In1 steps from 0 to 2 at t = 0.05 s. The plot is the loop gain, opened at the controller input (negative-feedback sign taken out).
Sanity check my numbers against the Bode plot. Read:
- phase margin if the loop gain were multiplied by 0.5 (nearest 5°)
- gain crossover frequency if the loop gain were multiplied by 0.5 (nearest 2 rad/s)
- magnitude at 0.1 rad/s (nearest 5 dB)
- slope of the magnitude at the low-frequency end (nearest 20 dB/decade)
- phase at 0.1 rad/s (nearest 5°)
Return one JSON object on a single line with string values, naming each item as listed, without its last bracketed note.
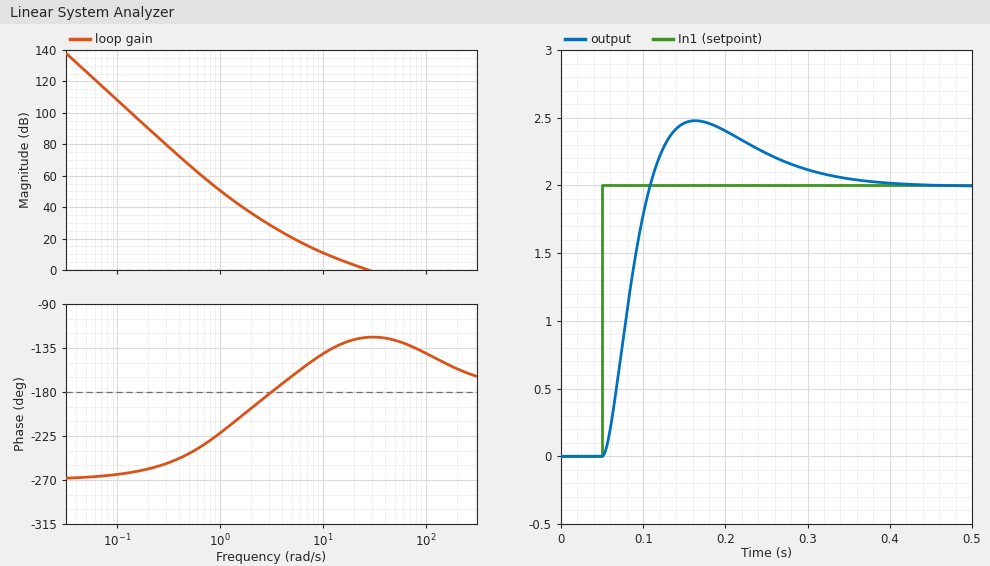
{"phase margin if the loop gain were multiplied by 0.5": "50°", "gain crossover frequency if the loop gain were multiplied by 0.5": "16 rad/s", "magnitude at 0.1 rad/s": "110 dB", "slope of the magnitude at the low-frequency end": "-60 dB/decade", "phase at 0.1 rad/s": "-265°"}
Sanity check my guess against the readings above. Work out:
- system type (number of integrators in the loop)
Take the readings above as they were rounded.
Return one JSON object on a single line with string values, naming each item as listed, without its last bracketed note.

{"system type": "3"}
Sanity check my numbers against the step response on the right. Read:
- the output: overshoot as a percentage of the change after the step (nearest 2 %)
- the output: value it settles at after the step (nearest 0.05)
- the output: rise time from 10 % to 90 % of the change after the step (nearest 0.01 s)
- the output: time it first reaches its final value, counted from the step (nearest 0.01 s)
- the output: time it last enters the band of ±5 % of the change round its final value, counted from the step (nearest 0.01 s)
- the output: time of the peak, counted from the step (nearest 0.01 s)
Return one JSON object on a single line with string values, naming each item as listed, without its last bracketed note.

{"the output: overshoot as a percentage of the change after the step": "24 %", "the output: value it settles at after the step": "2.00", "the output: rise time from 10 % to 90 % of the change after the step": "0.04 s", "the output: time it first reaches its final value, counted from the step": "0.06 s", "the output: time it last enters the band of ±5 % of the change round its final value, counted from the step": "0.26 s", "the output: time of the peak, counted from the step": "0.11 s"}
